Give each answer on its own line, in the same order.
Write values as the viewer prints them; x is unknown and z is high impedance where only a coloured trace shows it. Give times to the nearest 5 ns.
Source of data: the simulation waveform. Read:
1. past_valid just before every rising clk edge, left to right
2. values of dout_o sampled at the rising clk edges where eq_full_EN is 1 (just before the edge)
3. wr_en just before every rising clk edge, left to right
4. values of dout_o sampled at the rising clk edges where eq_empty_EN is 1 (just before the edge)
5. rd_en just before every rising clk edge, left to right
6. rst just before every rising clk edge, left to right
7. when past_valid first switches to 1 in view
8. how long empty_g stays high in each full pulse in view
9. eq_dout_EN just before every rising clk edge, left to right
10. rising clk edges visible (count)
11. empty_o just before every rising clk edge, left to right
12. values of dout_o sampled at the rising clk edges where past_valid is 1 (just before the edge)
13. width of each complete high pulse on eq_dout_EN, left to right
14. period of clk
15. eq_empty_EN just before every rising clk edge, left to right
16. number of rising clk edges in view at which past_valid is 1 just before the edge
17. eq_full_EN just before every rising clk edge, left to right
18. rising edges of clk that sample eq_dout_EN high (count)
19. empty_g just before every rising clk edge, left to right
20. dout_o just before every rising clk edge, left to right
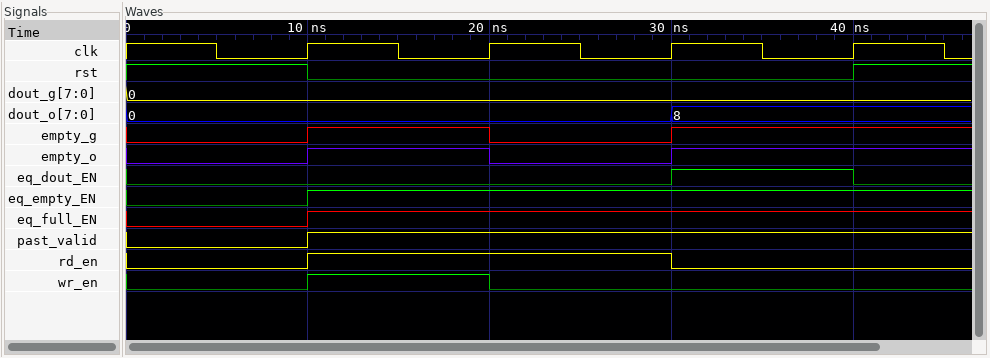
0 1 1 1
0, 0, 8
0 1 0 0
0, 0, 8
0 1 1 0
1 0 0 0
10 ns
10 ns
0 0 0 1
4
0 1 0 1
0, 0, 8
10 ns
10 ns
0 1 1 1
3
0 1 1 1
1
0 1 0 1
0, 0, 0, 8
